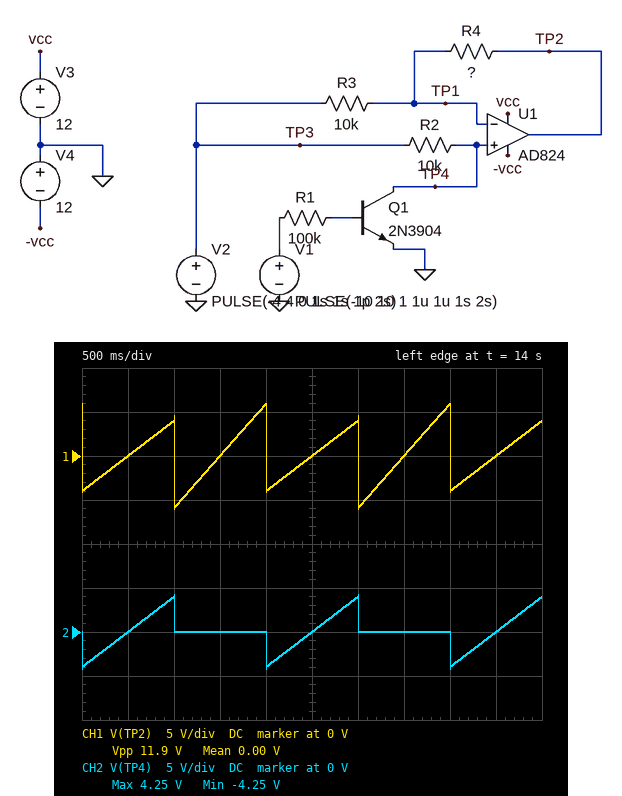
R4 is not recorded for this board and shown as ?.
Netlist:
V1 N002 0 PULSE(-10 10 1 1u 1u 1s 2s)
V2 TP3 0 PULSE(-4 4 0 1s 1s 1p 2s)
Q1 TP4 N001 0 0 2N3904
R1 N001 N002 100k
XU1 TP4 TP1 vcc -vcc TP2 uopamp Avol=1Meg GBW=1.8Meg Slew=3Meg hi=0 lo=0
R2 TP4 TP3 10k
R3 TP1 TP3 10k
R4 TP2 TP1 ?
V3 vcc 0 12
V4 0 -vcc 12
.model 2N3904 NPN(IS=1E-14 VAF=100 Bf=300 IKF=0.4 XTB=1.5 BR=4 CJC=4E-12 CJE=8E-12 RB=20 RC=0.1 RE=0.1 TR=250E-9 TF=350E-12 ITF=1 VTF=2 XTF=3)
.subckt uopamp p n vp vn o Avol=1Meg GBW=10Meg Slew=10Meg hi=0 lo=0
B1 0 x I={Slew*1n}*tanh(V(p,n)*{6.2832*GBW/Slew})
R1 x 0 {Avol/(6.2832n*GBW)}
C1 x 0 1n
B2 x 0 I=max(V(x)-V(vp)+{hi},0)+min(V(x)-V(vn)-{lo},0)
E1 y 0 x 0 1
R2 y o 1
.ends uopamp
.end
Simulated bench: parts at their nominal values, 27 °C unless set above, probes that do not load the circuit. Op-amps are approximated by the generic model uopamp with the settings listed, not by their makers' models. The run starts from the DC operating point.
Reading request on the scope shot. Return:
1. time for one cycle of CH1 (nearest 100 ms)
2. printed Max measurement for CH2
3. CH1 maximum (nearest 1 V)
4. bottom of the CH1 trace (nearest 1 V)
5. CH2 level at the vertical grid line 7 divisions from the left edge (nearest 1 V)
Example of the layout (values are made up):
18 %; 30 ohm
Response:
1.0 s; 4.25 V; 6 V; -6 V; 0 V
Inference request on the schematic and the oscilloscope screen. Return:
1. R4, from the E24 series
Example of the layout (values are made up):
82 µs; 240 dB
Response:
15 kΩ
